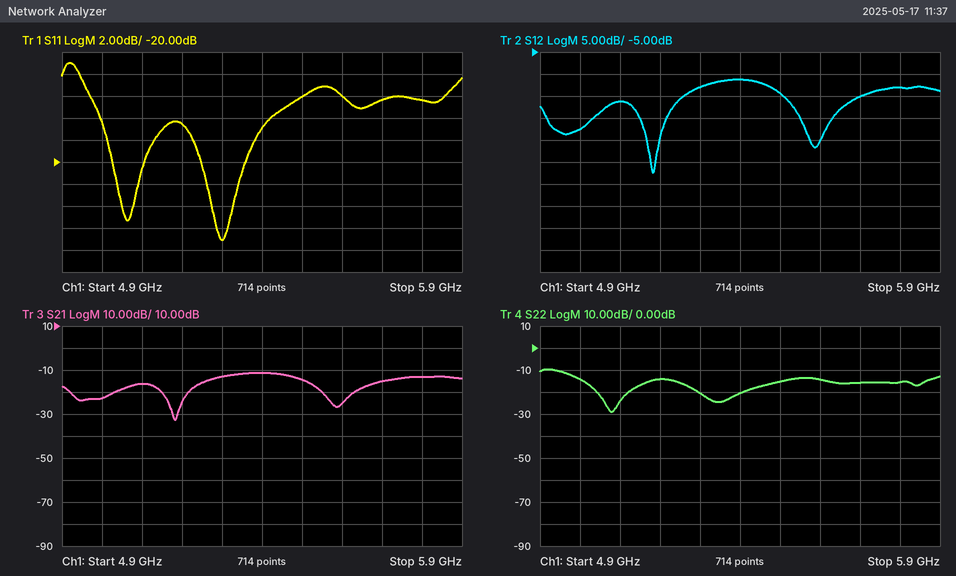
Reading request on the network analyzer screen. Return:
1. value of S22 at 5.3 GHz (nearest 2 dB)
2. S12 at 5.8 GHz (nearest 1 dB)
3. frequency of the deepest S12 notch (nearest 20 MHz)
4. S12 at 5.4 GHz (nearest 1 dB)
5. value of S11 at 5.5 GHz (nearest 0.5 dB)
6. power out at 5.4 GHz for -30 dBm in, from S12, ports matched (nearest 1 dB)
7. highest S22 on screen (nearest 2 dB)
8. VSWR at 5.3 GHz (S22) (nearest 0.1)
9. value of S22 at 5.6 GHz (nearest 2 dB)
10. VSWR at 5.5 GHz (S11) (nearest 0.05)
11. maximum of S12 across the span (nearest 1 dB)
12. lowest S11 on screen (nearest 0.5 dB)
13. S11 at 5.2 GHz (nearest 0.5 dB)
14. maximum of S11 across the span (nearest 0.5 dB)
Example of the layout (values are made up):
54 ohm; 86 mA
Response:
-20 dB; -13 dB; 5.18 GHz; -11 dB; -14.0 dB; -41 dBm; -10 dB; 1.2; -14 dB; 1.50; -11 dB; -27.0 dB; -16.5 dB; -11.0 dB
